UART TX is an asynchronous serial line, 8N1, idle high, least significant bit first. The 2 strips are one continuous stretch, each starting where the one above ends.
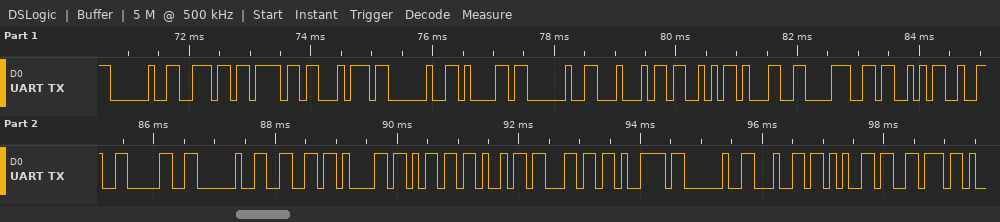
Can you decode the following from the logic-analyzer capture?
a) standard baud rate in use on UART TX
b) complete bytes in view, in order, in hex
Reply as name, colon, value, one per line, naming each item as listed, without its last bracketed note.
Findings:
standard baud rate in use on UART TX: 9600 baud
complete bytes in view, in order, in hex: 20 6E 6F 74 20 61 20 44 53 31 38 53 32 30 20 66 61 6D 69 6C 79 20 64 65 76
